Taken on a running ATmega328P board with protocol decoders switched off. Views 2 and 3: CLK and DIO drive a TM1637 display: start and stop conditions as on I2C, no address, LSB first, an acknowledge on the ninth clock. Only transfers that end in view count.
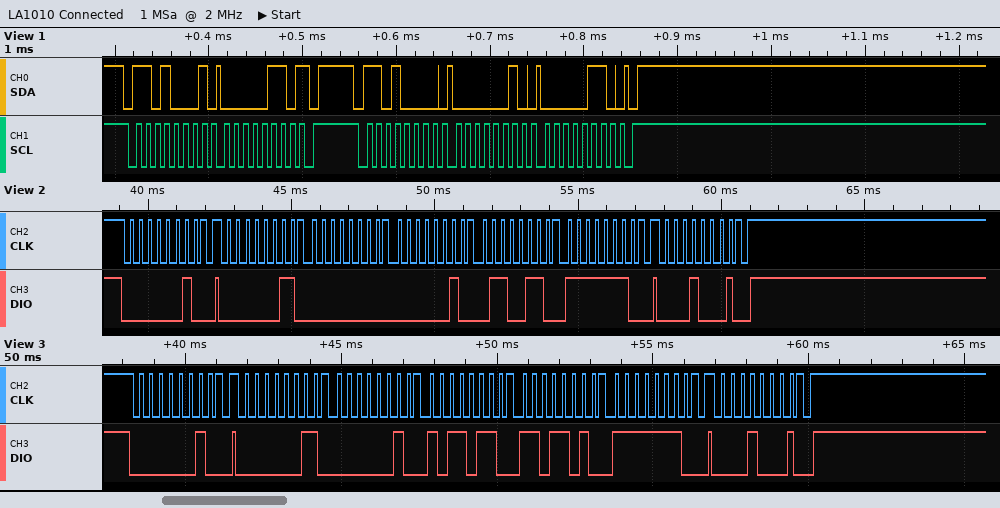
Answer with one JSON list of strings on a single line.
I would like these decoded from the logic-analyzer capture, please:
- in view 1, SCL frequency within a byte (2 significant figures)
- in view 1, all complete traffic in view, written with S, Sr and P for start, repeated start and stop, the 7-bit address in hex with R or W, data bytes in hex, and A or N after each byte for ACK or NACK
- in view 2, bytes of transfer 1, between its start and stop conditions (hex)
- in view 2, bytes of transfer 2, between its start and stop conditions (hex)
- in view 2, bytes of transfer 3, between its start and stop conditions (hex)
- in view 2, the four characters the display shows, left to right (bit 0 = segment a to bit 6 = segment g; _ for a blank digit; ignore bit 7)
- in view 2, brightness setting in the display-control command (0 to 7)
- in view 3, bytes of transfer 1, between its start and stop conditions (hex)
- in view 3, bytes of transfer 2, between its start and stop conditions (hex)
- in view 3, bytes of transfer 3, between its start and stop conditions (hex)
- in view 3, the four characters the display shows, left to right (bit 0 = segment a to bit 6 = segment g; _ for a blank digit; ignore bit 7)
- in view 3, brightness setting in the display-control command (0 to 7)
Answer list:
["100 kHz", "S 68R A 06 N P S 68W A 02 A 06 A P", "40", "C0 00 40 66 7F", "88", "_-48", "0", "40", "C0 40 6D 5B 7F", "88", "-528", "0"]
